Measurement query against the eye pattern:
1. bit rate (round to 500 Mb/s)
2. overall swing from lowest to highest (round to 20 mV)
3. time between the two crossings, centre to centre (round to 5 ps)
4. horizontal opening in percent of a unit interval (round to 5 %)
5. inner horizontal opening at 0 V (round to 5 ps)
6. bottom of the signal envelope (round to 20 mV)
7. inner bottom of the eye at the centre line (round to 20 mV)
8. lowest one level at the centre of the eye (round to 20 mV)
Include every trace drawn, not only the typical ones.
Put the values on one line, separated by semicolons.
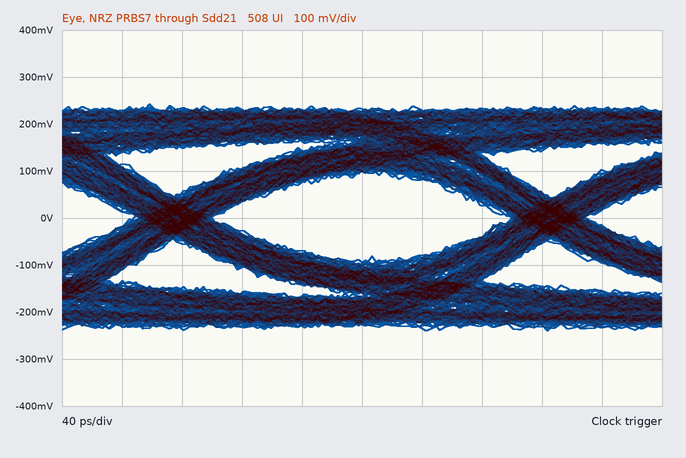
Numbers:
4.0 Gb/s; 480 mV; 250 ps; 80 %; 200 ps; -240 mV; -100 mV; 100 mV
